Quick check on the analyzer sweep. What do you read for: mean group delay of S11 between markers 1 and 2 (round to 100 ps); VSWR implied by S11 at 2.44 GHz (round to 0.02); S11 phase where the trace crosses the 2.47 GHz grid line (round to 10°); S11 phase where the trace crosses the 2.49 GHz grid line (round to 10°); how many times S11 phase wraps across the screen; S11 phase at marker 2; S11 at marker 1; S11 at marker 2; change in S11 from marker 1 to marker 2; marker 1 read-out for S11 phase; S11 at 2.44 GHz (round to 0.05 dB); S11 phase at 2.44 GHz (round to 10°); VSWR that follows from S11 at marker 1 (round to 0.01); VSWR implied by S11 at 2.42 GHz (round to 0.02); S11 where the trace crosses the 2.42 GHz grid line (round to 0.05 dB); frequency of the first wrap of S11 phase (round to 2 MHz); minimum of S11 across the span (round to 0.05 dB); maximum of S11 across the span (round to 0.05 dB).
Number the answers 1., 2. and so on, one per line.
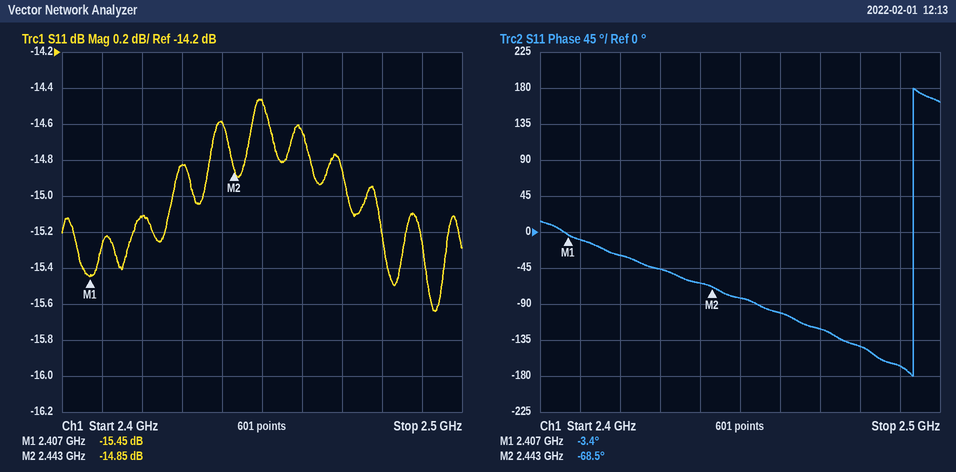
1. 5.0 ns
2. 1.46
3. -120°
4. -170°
5. 1
6. -68.5°
7. -15.45 dB
8. -14.85 dB
9. 0.60 dB
10. -3.4°
11. -14.60 dB
12. -60°
13. 1.41
14. 1.42
15. -15.10 dB
16. 2.494 GHz
17. -15.65 dB
18. -14.45 dB
